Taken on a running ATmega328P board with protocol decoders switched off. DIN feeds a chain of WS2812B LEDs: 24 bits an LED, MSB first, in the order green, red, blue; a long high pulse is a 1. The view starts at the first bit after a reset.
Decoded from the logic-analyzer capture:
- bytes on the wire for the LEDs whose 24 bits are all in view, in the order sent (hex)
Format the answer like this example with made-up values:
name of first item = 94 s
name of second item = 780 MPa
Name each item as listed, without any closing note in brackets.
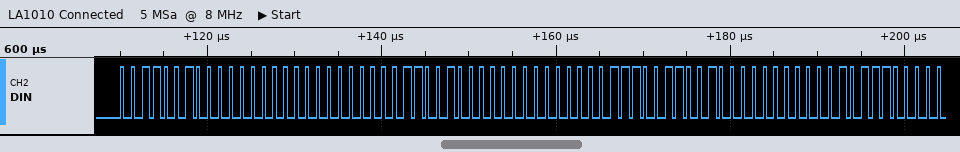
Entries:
bytes on the wire for the LEDs whose 24 bits are all in view, in the order sent = 32 00 00 32 00 07 32 00 2E
